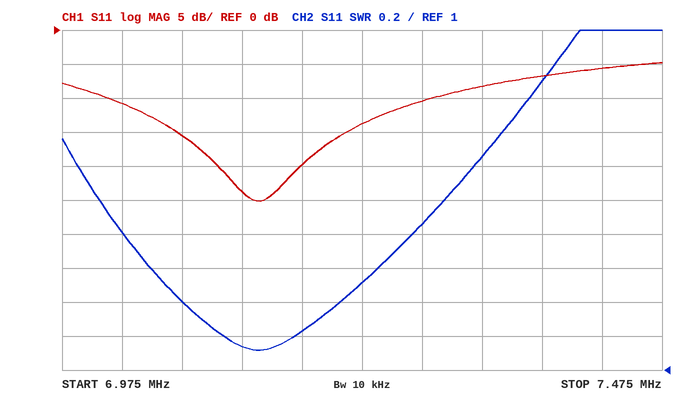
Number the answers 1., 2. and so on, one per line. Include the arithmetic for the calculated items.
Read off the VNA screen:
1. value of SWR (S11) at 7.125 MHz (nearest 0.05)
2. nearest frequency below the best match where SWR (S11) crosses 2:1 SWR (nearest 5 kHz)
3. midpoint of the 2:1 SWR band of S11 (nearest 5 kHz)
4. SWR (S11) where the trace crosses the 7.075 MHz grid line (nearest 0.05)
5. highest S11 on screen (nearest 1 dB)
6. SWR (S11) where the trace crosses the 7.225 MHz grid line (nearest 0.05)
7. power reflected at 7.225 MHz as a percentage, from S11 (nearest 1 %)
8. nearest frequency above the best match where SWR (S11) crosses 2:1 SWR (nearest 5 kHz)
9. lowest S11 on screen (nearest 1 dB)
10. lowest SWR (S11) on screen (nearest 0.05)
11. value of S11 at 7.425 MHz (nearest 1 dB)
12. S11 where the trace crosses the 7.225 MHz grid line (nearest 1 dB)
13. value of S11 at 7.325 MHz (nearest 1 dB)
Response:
1. 1.15
2. 7.005 MHz
3. 7.150 MHz
4. 1.40
5. -5 dB
6. 1.50
7. 10^(-14/10) ≈ 4 %
8. 7.295 MHz
9. -25 dB
10. 1.10
11. -6 dB
12. -14 dB
13. -8 dB
